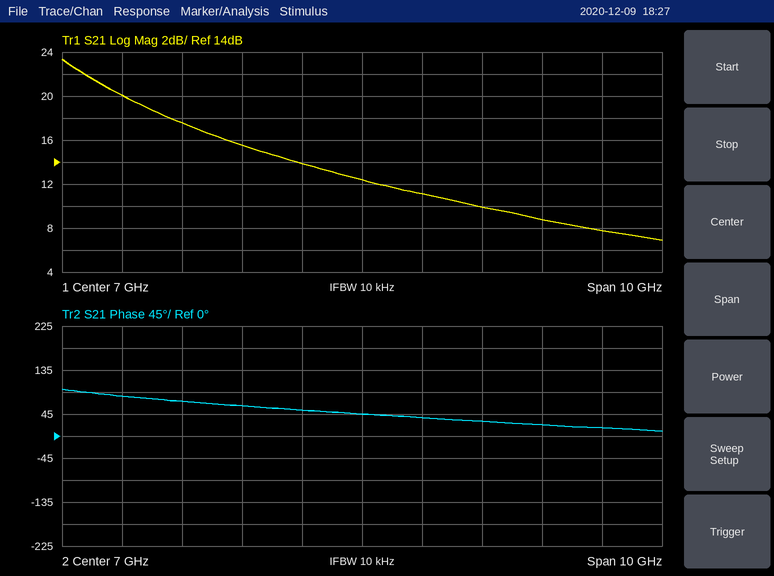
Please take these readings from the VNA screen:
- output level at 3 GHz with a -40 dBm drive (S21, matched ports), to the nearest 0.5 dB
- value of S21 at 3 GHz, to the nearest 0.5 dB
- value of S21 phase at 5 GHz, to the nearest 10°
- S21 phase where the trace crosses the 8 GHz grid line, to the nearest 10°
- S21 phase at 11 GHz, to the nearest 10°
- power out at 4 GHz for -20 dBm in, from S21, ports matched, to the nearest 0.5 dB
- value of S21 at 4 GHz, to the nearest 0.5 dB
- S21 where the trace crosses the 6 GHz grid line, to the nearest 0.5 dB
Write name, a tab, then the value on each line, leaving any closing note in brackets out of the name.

output level at 3 GHz with a -40 dBm drive (S21, matched ports), to the nearest 0.5 dB	-20.0 dBm
value of S21 at 3 GHz, to the nearest 0.5 dB	20.0 dB
value of S21 phase at 5 GHz, to the nearest 10°	60°
S21 phase where the trace crosses the 8 GHz grid line, to the nearest 10°	40°
S21 phase at 11 GHz, to the nearest 10°	20°
power out at 4 GHz for -20 dBm in, from S21, ports matched, to the nearest 0.5 dB	-2.5 dBm
value of S21 at 4 GHz, to the nearest 0.5 dB	17.5 dB
S21 where the trace crosses the 6 GHz grid line, to the nearest 0.5 dB	14.0 dB
